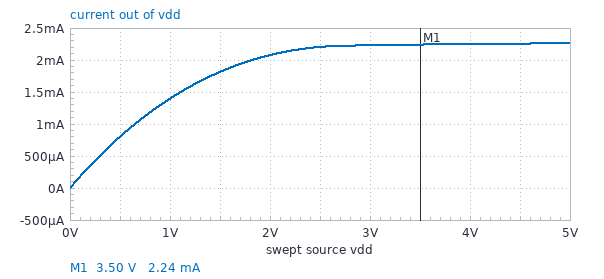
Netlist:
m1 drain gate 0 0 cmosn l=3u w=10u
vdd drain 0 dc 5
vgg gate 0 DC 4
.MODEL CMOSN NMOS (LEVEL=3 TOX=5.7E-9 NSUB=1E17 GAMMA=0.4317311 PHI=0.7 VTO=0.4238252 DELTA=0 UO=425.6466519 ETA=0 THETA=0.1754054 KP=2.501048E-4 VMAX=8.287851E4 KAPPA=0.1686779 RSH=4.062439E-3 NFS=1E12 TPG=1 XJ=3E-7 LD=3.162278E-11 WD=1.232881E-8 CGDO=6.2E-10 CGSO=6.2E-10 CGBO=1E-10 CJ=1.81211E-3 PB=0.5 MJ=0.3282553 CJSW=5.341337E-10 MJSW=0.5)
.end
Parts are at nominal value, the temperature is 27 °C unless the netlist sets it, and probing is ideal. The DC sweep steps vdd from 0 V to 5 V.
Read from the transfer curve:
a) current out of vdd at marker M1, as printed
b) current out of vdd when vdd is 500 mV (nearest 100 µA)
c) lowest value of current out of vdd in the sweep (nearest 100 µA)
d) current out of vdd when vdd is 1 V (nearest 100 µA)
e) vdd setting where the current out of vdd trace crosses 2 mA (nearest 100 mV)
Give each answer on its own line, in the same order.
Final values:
2.24 mA
800 µA
0 A
1.4 mA
1.8 V
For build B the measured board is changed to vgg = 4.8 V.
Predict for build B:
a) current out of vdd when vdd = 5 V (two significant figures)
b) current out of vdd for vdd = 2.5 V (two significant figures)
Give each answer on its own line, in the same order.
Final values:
3.0 mA
2.8 mA
